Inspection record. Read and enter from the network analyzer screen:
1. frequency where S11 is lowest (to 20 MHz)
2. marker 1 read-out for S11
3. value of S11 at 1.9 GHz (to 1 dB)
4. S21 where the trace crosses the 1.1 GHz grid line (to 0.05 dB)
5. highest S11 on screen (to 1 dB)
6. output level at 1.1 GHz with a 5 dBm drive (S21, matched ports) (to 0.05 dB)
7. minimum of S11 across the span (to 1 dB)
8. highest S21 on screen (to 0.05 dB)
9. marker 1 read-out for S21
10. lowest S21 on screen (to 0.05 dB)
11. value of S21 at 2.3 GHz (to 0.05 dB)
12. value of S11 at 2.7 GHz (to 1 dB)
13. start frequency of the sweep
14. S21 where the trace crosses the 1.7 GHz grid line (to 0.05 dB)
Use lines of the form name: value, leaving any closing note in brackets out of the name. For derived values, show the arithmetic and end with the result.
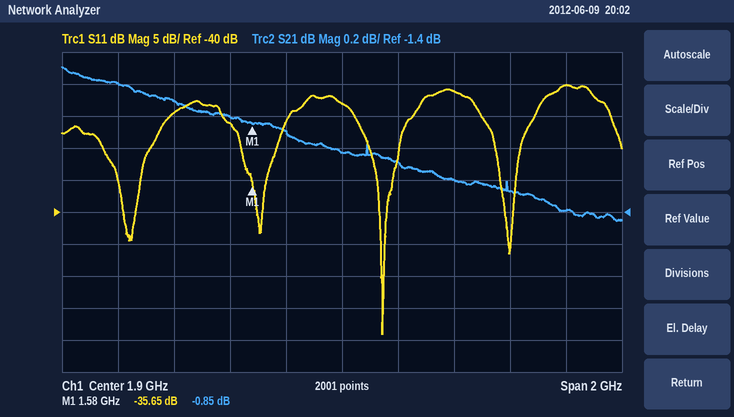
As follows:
frequency where S11 is lowest: 2.04 GHz
marker 1 read-out for S11: -35.65 dB
value of S11 at 1.9 GHz: -23 dB
S21 where the trace crosses the 1.1 GHz grid line: -0.60 dB
highest S11 on screen: -20 dB
output level at 1.1 GHz with a 5 dBm drive (S21, matched ports): 5 dBm + (-0.60 dB) = 4.40 dBm
minimum of S11 across the span: -59 dB
highest S21 on screen: -0.50 dB
marker 1 read-out for S21: -0.85 dB
lowest S21 on screen: -1.45 dB
value of S21 at 2.3 GHz: -1.20 dB
value of S11 at 2.7 GHz: -20 dB
start frequency of the sweep: 900 MHz
S21 where the trace crosses the 1.7 GHz grid line: -0.90 dB
